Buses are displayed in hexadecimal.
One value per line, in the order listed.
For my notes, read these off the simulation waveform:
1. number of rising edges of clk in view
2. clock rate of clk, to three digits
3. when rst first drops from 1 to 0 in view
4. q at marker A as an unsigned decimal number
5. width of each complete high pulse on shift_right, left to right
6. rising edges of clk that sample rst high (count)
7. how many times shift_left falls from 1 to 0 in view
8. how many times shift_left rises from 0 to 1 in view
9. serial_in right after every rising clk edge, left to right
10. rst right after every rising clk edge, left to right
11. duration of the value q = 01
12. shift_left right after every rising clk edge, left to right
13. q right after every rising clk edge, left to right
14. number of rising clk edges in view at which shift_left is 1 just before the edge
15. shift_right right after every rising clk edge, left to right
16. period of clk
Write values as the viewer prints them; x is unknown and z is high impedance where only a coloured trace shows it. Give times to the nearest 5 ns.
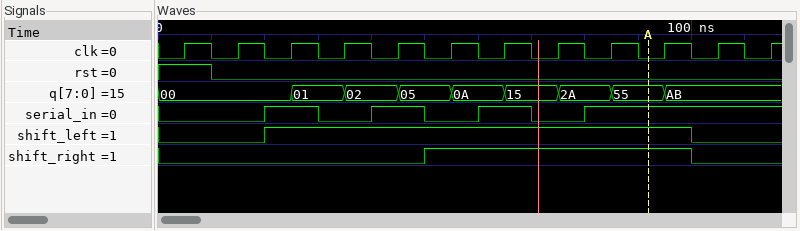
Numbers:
12
100 MHz
10 ns
85
50 ns
1
1
1
0 0 1 0 1 0 1 0 1 1 1 1
1 0 0 0 0 0 0 0 0 0 0 0
10 ns
0 0 1 1 1 1 1 1 1 1 0 0
00, 00, 01, 02, 05, 0A, 15, 2A, 55, AB, AB, AB
8
0 0 0 0 0 1 1 1 1 1 0 0
10 ns
